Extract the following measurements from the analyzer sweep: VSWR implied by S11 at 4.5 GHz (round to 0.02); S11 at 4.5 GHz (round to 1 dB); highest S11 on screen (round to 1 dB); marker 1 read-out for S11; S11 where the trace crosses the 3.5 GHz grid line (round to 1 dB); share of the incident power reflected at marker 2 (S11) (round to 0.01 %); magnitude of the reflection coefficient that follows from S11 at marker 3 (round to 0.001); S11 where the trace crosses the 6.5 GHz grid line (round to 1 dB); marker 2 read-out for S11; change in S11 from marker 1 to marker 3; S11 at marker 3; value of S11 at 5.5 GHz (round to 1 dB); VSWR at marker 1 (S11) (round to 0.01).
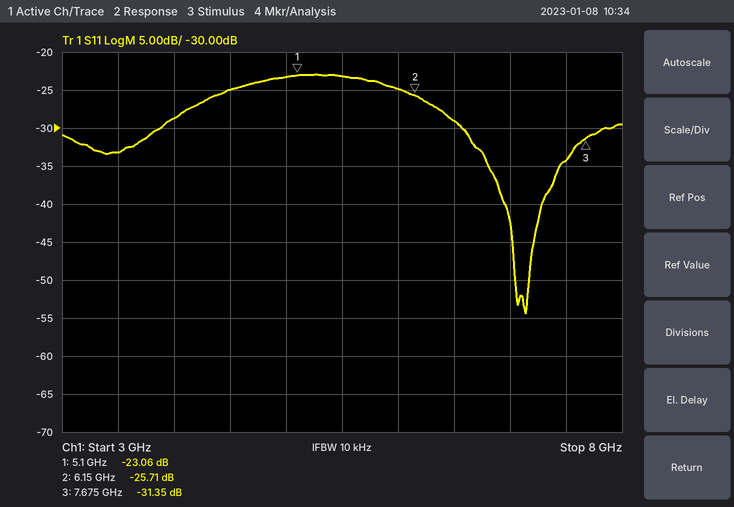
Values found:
1.12
-25 dB
-23 dB
-23.06 dB
-33 dB
0.27 %
0.027
-29 dB
-25.71 dB
-8.29 dB
-31.35 dB
-23 dB
1.15
